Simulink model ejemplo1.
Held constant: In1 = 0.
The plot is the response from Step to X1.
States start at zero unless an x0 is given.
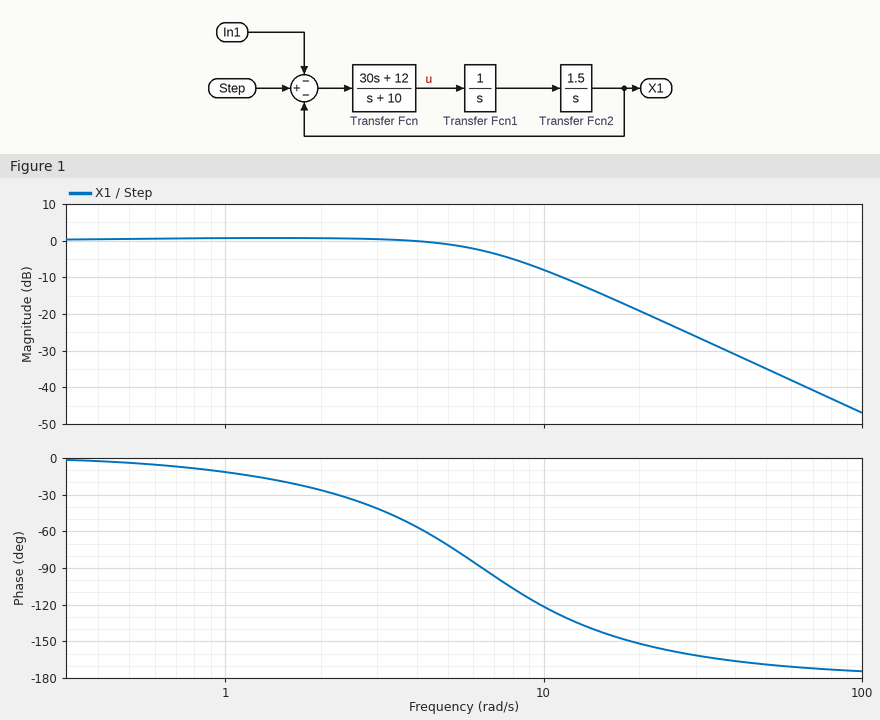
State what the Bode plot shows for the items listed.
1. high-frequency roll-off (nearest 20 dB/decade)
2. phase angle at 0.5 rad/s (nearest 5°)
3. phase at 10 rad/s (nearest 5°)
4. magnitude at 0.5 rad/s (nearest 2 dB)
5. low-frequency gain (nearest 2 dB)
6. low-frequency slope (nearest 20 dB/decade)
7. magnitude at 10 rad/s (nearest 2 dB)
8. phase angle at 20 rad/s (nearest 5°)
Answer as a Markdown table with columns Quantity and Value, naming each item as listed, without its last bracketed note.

| Quantity | Value |
|---|---|
| high-frequency roll-off | -40 dB/decade |
| phase angle at 0.5 rad/s | -5° |
| phase at 10 rad/s | -120° |
| magnitude at 0.5 rad/s | 0 dB |
| low-frequency gain | 0 dB |
| low-frequency slope | 0 dB/decade |
| magnitude at 10 rad/s | -8 dB |
| phase angle at 20 rad/s | -150° |
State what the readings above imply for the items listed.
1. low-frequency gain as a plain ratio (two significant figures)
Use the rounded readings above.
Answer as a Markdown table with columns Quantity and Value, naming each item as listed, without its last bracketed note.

| Quantity | Value |
|---|---|
| low-frequency gain as a plain ratio | 1.0 |
